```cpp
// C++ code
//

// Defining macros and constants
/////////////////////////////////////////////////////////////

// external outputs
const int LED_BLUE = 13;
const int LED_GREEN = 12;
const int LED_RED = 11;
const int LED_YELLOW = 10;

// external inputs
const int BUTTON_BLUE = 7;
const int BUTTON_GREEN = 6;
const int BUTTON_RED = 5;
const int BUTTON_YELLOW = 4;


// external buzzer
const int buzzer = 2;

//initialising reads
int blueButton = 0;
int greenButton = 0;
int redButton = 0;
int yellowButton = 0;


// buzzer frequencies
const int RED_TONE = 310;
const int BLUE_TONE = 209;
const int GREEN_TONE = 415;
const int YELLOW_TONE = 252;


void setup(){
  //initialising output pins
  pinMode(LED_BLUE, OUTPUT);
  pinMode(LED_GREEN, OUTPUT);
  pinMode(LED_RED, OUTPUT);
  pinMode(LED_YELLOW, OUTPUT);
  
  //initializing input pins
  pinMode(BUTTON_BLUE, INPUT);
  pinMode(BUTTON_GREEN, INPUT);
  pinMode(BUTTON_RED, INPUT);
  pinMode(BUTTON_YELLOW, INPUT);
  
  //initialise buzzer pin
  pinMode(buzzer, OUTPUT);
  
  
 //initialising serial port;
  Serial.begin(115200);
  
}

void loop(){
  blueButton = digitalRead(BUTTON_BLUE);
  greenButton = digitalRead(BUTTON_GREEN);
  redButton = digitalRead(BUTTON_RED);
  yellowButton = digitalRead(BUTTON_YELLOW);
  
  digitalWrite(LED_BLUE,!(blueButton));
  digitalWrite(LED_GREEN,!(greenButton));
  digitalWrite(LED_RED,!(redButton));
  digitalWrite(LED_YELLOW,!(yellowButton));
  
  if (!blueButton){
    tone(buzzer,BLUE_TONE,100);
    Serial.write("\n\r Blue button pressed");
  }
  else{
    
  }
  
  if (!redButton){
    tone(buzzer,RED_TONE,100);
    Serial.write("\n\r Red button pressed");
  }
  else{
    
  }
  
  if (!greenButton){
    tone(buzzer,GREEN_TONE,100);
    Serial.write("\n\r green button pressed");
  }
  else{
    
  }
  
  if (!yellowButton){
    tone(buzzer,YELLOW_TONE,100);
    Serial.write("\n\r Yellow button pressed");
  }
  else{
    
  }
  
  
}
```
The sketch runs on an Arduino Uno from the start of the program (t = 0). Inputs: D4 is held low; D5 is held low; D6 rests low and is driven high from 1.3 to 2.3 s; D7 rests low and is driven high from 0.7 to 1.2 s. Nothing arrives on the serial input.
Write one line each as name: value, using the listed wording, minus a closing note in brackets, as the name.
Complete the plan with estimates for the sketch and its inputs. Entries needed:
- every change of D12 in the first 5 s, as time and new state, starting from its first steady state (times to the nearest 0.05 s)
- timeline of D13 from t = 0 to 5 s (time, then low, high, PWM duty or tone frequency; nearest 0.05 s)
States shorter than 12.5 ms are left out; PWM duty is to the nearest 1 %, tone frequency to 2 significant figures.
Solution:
every change of D12 in the first 5 s, as time and new state, starting from its first steady state: 0 s high; 1.3 s low; 2.3 s high
timeline of D13 from t = 0 to 5 s: 0 s high; 0.7 s low; 1.2 s high
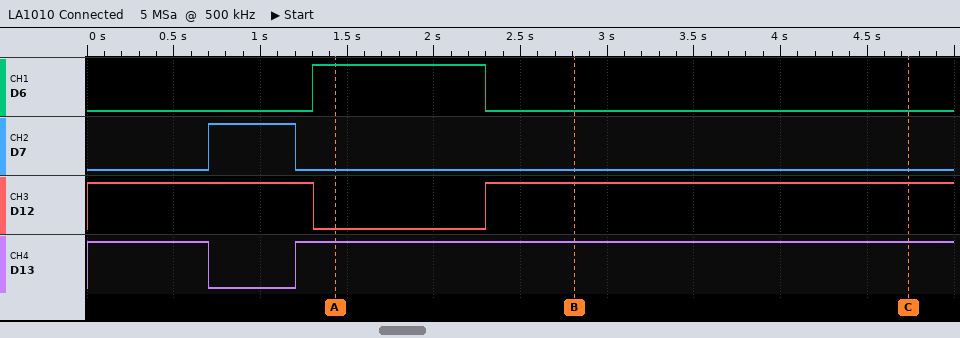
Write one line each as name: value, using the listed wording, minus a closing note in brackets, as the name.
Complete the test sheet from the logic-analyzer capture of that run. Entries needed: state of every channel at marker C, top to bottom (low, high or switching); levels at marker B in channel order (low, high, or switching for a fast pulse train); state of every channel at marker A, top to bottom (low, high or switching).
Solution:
state of every channel at marker C, top to bottom: D6 low, D7 low, D12 high, D13 high
levels at marker B in channel order: D6 low, D7 low, D12 high, D13 high
state of every channel at marker A, top to bottom: D6 high, D7 low, D12 low, D13 high
